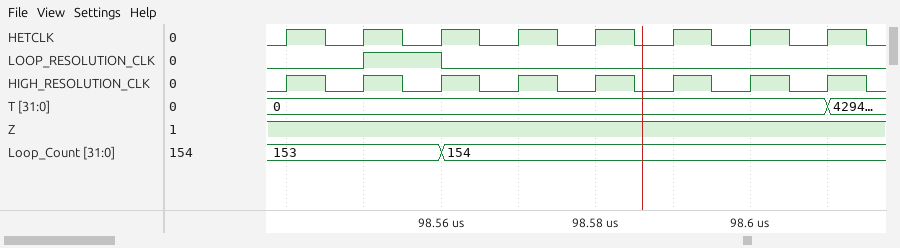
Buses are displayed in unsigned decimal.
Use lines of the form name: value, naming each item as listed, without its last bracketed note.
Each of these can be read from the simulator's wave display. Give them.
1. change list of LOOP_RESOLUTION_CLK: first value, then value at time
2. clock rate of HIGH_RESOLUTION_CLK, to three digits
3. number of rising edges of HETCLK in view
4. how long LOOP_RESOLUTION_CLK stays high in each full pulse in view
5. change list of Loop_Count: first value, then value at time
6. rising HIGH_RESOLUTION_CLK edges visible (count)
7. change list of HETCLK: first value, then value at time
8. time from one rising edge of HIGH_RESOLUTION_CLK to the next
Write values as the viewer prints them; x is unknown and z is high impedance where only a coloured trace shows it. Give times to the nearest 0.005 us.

change list of LOOP_RESOLUTION_CLK: first value, then value at time: 0, 1 at 98.55 us, 0 at 98.56 us
clock rate of HIGH_RESOLUTION_CLK, to three digits: 100 MHz
number of rising edges of HETCLK in view: 8
how long LOOP_RESOLUTION_CLK stays high in each full pulse in view: 0.01 us
change list of Loop_Count: first value, then value at time: 153, 154 at 98.56 us
rising HIGH_RESOLUTION_CLK edges visible: 8
change list of HETCLK: first value, then value at time: 0, 1 at 98.54 us, 0 at 98.545 us, 1 at 98.55 us, 0 at 98.555 us, 1 at 98.56 us, 0 at 98.565 us, 1 at 98.57 us, 0 at 98.575 us, 1 at 98.58 us, 0 at 98.585 us, 1 at 98.59 us, 0 at 98.595 us, 1 at 98.6 us, 0 at 98.605 us, 1 at 98.61 us, 0 at 98.615 us
time from one rising edge of HIGH_RESOLUTION_CLK to the next: 0.01 us
